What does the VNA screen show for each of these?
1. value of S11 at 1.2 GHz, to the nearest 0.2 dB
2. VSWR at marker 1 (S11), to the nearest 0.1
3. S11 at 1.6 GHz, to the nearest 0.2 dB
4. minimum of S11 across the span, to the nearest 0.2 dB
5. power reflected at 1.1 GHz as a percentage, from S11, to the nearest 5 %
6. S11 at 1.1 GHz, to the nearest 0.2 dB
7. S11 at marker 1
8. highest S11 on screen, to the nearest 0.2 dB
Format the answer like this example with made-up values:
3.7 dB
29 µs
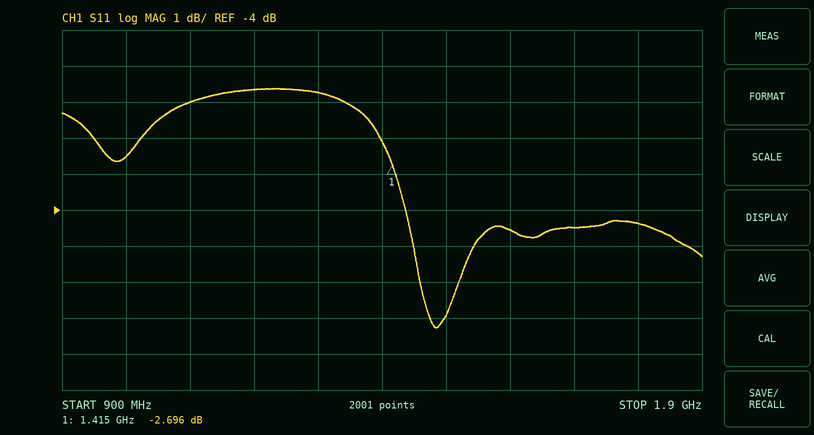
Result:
-0.6 dB
6.5
-4.6 dB
-7.2 dB
80 %
-1.0 dB
-2.696 dB
-0.6 dB
